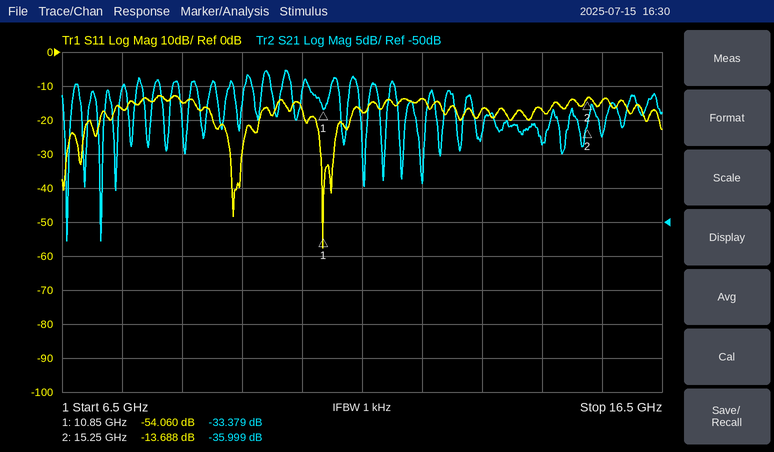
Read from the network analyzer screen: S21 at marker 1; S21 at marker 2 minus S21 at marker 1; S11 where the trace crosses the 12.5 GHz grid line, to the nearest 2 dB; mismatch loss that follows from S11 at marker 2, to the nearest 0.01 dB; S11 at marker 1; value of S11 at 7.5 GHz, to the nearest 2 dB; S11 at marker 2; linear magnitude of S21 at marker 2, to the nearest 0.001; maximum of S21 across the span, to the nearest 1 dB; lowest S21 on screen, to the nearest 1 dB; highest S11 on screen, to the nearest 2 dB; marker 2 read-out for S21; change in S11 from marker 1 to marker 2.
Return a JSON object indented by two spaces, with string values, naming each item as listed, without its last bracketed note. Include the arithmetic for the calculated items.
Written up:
{
  "S21 at marker 1": "-33.379 dB",
  "S21 at marker 2 minus S21 at marker 1": "-35.999 − (-33.379) = -2.620 dB",
  "S11 where the trace crosses the 12.5 GHz grid line, to the nearest 2 dB": "-14 dB",
  "mismatch loss that follows from S11 at marker 2, to the nearest 0.01 dB": "−10 log10(1 − 10^(-13.688/10)) ≈ 0.19 dB",
  "S11 at marker 1": "-54.060 dB",
  "value of S11 at 7.5 GHz, to the nearest 2 dB": "-16 dB",
  "S11 at marker 2": "-13.688 dB",
  "linear magnitude of S21 at marker 2, to the nearest 0.001": "10^(-35.999/20) ≈ 0.016",
  "maximum of S21 across the span, to the nearest 1 dB": "-28 dB",
  "lowest S21 on screen, to the nearest 1 dB": "-53 dB",
  "highest S11 on screen, to the nearest 2 dB": "-12 dB",
  "marker 2 read-out for S21": "-35.999 dB",
  "change in S11 from marker 1 to marker 2": "-13.688 − (-54.06) = 40.372 dB"
}
